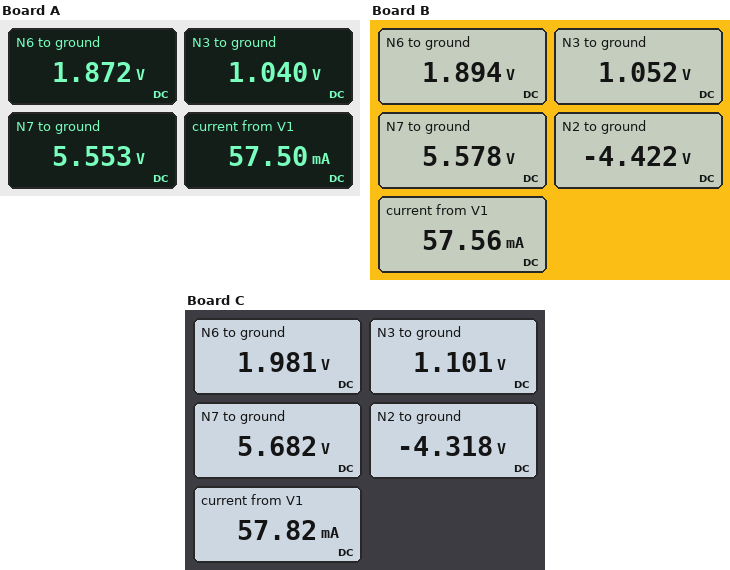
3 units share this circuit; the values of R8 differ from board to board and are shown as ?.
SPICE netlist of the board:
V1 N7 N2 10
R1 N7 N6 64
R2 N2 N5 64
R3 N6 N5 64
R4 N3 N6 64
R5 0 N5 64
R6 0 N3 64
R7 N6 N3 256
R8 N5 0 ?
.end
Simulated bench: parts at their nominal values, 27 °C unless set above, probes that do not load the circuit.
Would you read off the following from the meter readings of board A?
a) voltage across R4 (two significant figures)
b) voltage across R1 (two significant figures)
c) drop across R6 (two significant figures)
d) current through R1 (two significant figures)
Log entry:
830 mV
3.7 V
1.0 V
58 mA
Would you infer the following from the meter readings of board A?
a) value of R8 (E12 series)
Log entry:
180 Ω
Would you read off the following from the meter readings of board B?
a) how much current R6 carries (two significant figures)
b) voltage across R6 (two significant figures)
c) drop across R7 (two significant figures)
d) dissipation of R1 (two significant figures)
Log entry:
16 mA
1.1 V
840 mV
210 mW
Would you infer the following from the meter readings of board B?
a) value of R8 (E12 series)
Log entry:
150 Ω
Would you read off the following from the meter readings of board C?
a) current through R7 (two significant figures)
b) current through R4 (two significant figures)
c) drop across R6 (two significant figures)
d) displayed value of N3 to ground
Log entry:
3.4 mA
14 mA
1.1 V
1.101 V
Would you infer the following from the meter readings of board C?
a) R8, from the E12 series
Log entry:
82 Ω
